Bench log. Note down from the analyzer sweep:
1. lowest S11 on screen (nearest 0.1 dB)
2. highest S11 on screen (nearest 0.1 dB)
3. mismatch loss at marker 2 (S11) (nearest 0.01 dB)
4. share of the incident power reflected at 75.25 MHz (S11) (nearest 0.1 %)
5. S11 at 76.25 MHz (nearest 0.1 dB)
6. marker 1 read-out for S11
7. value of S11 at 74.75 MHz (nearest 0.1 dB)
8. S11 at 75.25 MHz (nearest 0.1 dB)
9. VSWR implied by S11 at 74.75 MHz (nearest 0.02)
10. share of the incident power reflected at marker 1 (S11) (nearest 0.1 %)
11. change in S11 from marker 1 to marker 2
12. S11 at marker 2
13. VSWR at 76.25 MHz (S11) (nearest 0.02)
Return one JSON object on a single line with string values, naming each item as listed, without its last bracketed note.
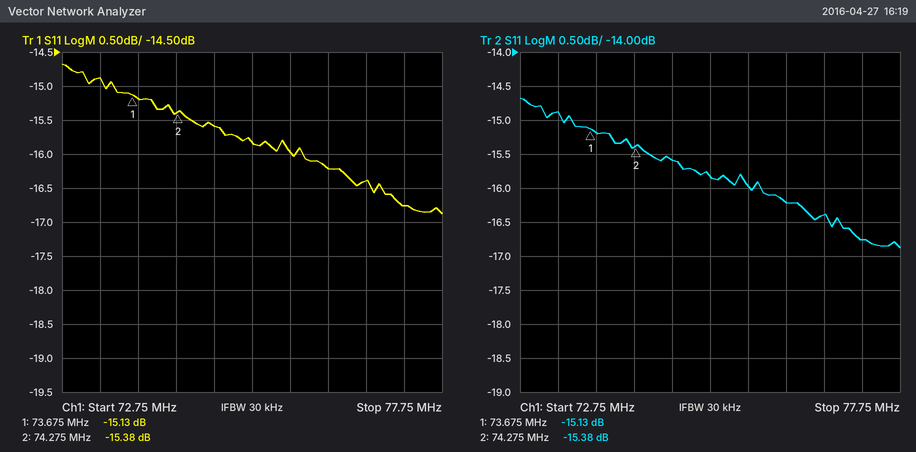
{"lowest S11 on screen": "-16.9 dB", "highest S11 on screen": "-14.7 dB", "mismatch loss at marker 2 (S11)": "0.13 dB", "share of the incident power reflected at 75.25 MHz (S11)": "2.6 %", "S11 at 76.25 MHz": "-16.2 dB", "marker 1 read-out for S11": "-15.13 dB", "value of S11 at 74.75 MHz": "-15.6 dB", "S11 at 75.25 MHz": "-15.8 dB", "VSWR implied by S11 at 74.75 MHz": "1.40", "share of the incident power reflected at marker 1 (S11)": "3.1 %", "change in S11 from marker 1 to marker 2": "-0.25 dB", "S11 at marker 2": "-15.38 dB", "VSWR at 76.25 MHz (S11)": "1.36"}
